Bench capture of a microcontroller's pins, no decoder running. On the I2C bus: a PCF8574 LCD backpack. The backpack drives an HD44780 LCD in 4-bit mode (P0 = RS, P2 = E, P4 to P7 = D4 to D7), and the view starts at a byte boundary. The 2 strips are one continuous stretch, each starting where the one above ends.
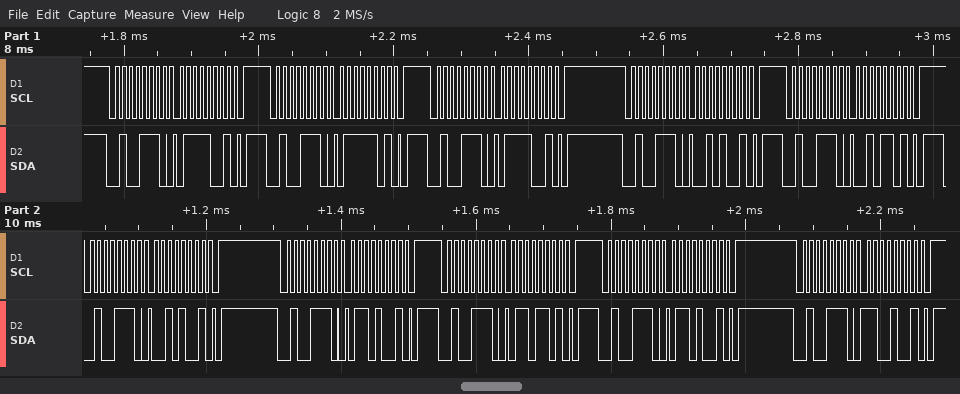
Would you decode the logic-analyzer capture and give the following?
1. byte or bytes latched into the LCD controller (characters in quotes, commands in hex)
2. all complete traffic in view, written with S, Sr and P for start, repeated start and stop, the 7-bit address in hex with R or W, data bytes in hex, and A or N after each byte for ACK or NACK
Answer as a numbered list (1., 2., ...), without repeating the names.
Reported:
1. 'r'
2. S 27W A 79 A P S 27W A 7D A P S 27W A 79 A P S 27W A 29 A P S 27W A 2D A P S 27W A 29 A P S 27W A 69 A P S 27W A 6D A P S 27W A 69 A P S 27W A C9 A P
